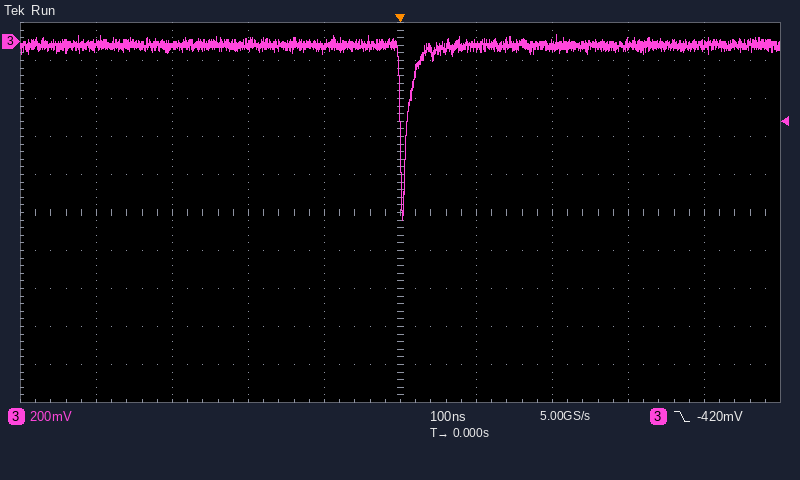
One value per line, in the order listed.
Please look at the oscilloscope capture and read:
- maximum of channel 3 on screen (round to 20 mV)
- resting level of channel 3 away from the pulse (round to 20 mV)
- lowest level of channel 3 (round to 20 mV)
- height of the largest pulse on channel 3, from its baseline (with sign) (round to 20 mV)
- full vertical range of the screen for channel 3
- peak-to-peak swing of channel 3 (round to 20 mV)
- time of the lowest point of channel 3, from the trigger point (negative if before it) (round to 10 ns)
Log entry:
40 mV
-20 mV
-940 mV
-920 mV
2 V
980 mV
0 ns
